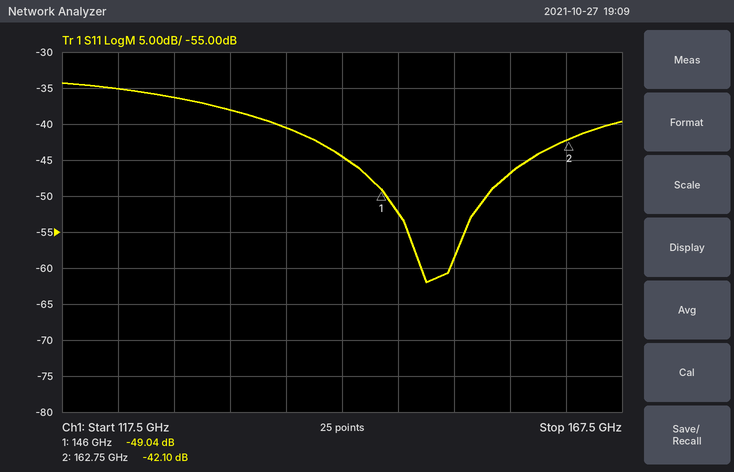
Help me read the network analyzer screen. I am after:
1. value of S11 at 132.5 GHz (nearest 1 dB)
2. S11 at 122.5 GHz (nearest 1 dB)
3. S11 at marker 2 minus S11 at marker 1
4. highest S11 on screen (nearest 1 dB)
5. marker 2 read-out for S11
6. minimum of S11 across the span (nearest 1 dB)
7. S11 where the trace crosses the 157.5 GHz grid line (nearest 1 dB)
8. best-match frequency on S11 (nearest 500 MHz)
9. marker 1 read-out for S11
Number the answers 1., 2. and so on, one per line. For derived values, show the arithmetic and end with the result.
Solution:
1. -38 dB
2. -35 dB
3. -42.1 − (-49.04) = 6.94 dB
4. -34 dB
5. -42.10 dB
6. -62 dB
7. -47 dB
8. 150.0 GHz
9. -49.04 dB
